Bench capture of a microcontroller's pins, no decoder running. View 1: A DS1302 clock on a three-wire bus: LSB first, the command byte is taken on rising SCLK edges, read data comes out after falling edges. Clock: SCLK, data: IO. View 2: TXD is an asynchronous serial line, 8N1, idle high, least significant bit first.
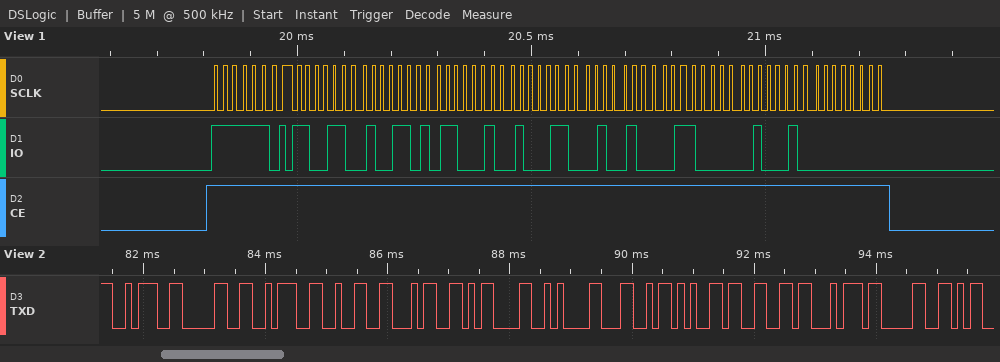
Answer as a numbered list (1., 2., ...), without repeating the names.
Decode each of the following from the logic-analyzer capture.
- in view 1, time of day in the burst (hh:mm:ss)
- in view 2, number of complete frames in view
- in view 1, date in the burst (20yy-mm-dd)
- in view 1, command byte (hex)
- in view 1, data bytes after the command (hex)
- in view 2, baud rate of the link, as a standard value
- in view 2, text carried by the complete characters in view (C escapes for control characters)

1. 23:59:33
2. 12
3. 2022-12-31
4. 0xBF
5. 33 59 23 31 12 06 22 00
6. 9600 baud
7. ":0:24\r\nLeft0"
